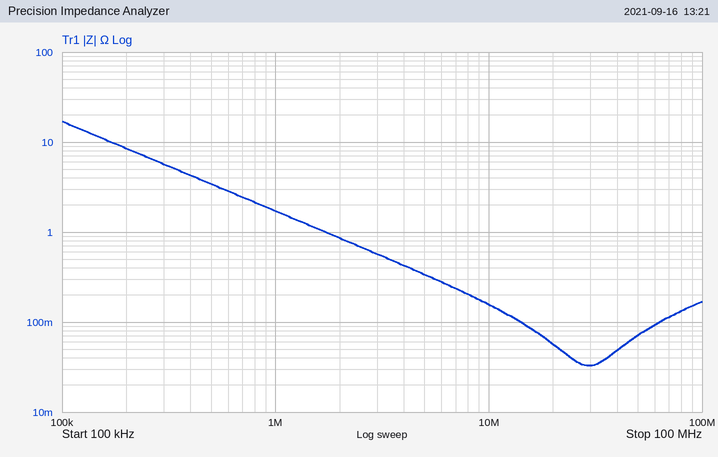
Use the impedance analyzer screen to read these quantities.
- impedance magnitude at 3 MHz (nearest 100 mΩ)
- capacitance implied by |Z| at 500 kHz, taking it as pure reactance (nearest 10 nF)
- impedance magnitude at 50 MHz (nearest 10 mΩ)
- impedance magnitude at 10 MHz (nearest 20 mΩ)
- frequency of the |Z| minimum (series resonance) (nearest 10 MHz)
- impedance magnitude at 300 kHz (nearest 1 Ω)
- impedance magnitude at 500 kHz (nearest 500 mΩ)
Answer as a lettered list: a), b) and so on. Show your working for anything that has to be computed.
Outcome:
a) 600 mΩ
b) C = 1/(2π × 500 kHz × 3.5 Ω) ≈ 90.9 nF, so 90 nF to the nearest 10 nF
c) 70 mΩ
d) 160 mΩ
e) 30 MHz
f) 6 Ω
g) 3.5 Ω
